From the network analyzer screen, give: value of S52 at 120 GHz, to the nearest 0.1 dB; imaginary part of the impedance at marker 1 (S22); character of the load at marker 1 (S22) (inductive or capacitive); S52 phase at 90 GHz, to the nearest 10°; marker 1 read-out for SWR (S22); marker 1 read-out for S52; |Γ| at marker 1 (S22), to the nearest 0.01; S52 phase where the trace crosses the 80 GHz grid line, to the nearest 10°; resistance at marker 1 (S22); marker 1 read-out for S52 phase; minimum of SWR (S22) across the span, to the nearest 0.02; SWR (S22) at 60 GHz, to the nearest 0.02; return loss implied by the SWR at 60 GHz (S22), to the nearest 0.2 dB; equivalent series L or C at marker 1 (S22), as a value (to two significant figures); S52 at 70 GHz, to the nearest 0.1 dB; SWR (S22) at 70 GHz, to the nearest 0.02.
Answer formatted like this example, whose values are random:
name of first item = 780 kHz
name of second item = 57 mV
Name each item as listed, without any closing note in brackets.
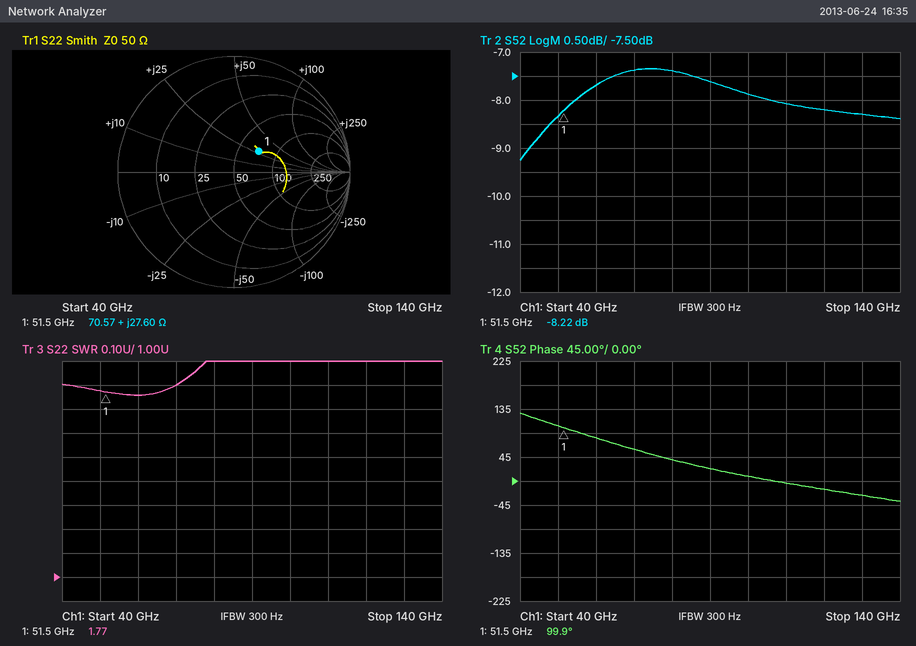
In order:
value of S52 at 120 GHz, to the nearest 0.1 dB = -8.2 dB
imaginary part of the impedance at marker 1 = +27.60 Ω
character of the load at marker 1 (S22) = inductive
S52 phase at 90 GHz, to the nearest 10° = 20°
marker 1 read-out for SWR = 1.77
marker 1 read-out for S52 = -8.22 dB
|Γ| at marker 1 (S22), to the nearest 0.01 = 0.28
S52 phase where the trace crosses the 80 GHz grid line, to the nearest 10° = 40°
resistance at marker 1 = 70.57 Ω
marker 1 read-out for S52 phase = 99.9°
minimum of SWR (S22) across the span, to the nearest 0.02 = 1.76
SWR (S22) at 60 GHz, to the nearest 0.02 = 1.76
return loss implied by the SWR at 60 GHz (S22), to the nearest 0.2 dB = 11.2 dB
equivalent series L or C at marker 1 (S22), as a value = 85 pH
S52 at 70 GHz, to the nearest 0.1 dB = -7.4 dB
SWR (S22) at 70 GHz, to the nearest 0.02 = 1.80
